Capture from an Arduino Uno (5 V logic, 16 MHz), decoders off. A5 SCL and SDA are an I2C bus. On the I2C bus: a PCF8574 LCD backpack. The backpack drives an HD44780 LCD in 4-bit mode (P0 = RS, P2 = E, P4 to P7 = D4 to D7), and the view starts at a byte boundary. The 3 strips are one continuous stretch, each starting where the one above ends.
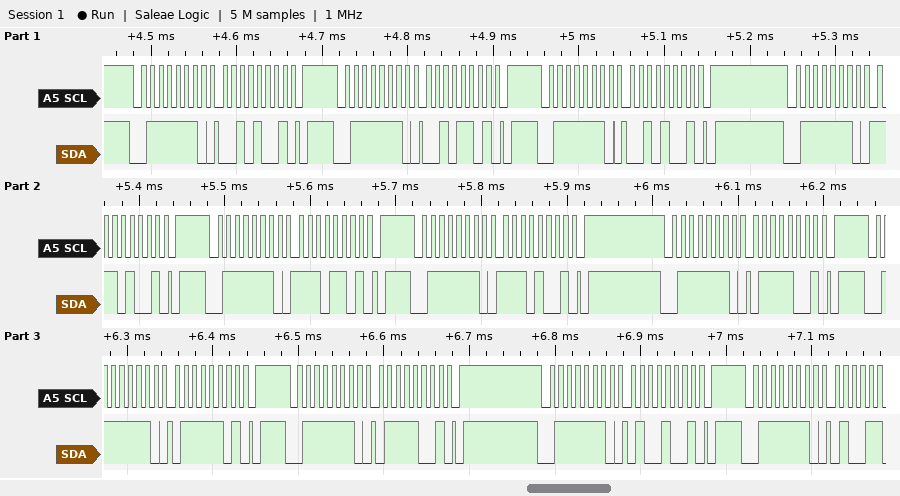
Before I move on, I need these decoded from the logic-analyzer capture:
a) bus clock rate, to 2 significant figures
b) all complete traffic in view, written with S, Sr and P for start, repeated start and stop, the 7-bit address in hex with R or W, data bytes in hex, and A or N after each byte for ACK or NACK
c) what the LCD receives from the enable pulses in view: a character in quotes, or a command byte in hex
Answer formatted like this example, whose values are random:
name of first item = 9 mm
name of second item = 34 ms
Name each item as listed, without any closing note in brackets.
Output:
bus clock rate, to 2 significant figures = 100 kHz
all complete traffic in view, written with S, Sr and P for start, repeated start and stop, the 7-bit address in hex with R or W, data bytes in hex, and A or N after each byte for ACK or NACK = S 3FW A 29 A P S 3FW A 2D A P S 3FW A 29 A P S 3FW A E9 A P S 3FW A ED A P S 3FW A E9 A P S 3FW A 79 A P S 3FW A 7D A P S 3FW A 79 A P S 3FW A 49 A P S 3FW A
what the LCD receives from the enable pulses in view: a character in quotes, or a command byte in hex = '.'
